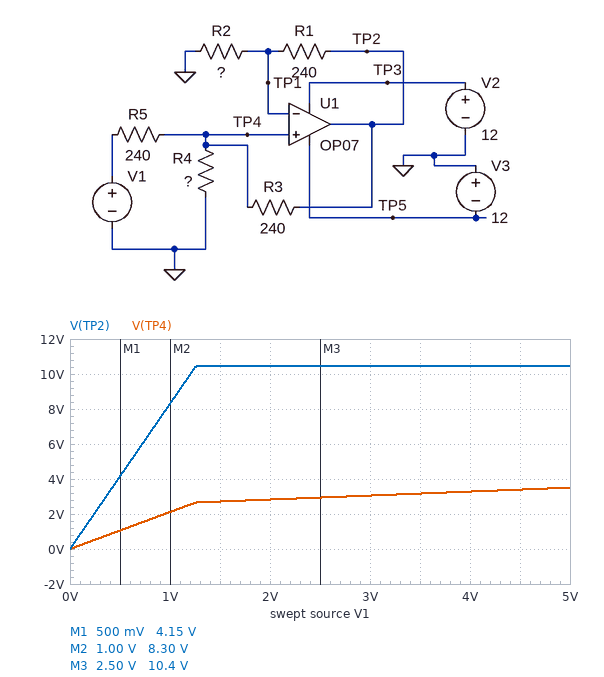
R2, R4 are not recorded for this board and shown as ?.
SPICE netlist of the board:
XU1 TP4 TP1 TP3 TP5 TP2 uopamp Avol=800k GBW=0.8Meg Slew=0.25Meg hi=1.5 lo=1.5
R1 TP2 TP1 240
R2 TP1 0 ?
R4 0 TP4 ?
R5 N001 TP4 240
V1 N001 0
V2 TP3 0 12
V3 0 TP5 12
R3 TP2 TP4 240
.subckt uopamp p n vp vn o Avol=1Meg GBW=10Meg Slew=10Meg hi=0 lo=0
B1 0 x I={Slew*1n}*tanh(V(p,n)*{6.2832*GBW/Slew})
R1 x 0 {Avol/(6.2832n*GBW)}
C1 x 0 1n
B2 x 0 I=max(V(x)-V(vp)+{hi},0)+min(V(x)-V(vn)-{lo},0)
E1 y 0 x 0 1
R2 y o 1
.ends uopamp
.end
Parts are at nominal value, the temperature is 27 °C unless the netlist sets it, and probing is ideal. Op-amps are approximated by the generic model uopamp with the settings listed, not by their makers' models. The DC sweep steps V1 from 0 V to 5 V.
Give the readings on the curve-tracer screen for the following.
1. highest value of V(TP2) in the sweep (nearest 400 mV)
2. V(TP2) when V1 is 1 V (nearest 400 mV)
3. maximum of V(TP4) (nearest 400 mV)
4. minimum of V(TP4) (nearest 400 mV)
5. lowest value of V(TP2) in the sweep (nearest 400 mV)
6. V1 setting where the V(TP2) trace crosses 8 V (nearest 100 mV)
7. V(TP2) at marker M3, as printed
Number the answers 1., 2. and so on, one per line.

1. 10.4 V
2. 8.4 V
3. 3.6 V
4. 0 V
5. 0 V
6. 1.0 V
7. 10.4 V
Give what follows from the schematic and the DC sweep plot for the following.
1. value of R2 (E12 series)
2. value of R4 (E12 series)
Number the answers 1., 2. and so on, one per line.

1. 82 Ω
2. 100 Ω
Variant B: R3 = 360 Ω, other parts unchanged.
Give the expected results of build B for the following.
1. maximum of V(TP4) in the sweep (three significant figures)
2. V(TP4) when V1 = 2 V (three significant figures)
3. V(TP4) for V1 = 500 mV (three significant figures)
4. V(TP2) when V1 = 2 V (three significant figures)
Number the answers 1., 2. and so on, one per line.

1. 2.94 V
2. 1.38 V
3. 345 mV
4. 5.42 V
